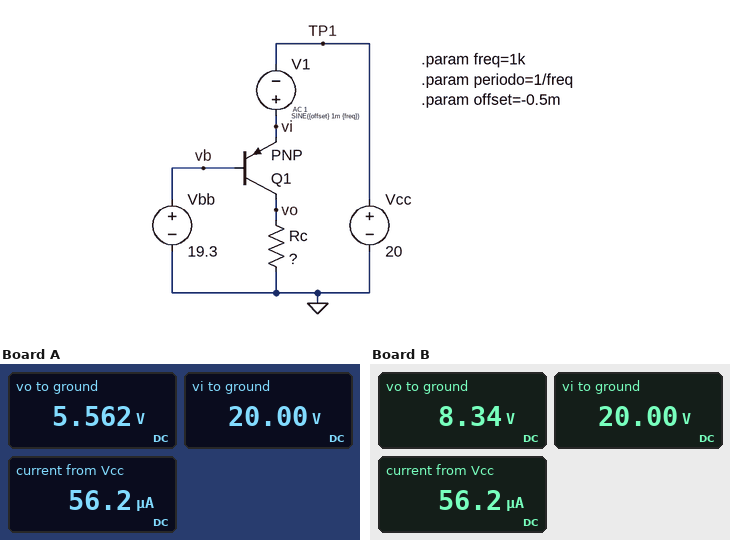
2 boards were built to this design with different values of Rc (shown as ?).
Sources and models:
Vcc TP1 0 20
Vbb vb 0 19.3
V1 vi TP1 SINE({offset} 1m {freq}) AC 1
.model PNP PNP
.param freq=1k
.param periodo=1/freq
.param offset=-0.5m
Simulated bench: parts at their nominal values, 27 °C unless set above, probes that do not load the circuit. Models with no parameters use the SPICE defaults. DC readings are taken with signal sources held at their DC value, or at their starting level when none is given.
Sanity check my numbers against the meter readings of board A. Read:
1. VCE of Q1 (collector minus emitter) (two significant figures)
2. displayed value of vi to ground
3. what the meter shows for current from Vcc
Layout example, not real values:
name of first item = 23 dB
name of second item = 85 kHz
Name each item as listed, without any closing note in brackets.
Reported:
VCE of Q1 (collector minus emitter) = -14 V
displayed value of vi to ground = 20.00 V
what the meter shows for current from Vcc = 56.2 µA
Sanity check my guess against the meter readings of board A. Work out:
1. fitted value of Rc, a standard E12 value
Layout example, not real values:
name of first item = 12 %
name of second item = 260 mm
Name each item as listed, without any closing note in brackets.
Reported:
fitted value of Rc, a standard E12 value = 100 kΩ
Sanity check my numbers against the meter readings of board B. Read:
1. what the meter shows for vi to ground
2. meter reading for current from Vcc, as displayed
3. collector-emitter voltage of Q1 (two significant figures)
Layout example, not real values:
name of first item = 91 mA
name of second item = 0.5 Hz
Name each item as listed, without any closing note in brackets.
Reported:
what the meter shows for vi to ground = 20.00 V
meter reading for current from Vcc, as displayed = 56.2 µA
collector-emitter voltage of Q1 = -12 V
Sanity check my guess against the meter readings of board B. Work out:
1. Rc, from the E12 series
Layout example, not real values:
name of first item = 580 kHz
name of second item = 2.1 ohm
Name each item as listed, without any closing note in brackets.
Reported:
Rc, from the E12 series = 150 kΩ
